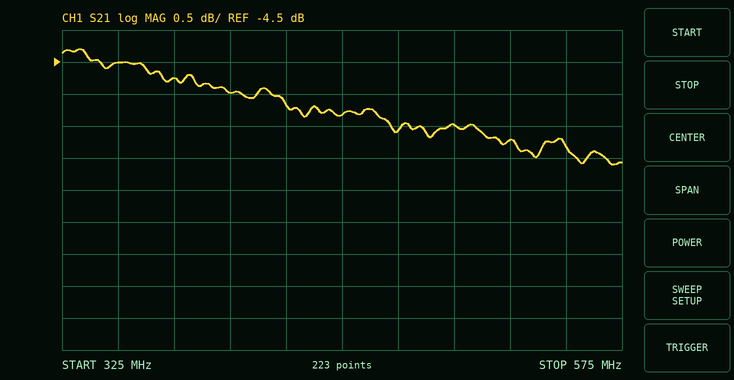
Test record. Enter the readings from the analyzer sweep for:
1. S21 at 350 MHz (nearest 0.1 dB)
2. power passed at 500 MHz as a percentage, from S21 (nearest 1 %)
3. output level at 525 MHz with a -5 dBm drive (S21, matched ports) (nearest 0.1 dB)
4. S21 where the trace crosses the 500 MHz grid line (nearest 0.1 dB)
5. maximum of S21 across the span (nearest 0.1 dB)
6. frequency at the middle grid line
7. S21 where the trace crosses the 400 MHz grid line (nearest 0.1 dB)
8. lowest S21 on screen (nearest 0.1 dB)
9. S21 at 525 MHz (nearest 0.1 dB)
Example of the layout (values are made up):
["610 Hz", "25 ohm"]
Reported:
["-4.5 dB", "28 %", "-10.7 dBm", "-5.5 dB", "-4.3 dB", "450 MHz", "-5.0 dB", "-6.1 dB", "-5.7 dB"]
